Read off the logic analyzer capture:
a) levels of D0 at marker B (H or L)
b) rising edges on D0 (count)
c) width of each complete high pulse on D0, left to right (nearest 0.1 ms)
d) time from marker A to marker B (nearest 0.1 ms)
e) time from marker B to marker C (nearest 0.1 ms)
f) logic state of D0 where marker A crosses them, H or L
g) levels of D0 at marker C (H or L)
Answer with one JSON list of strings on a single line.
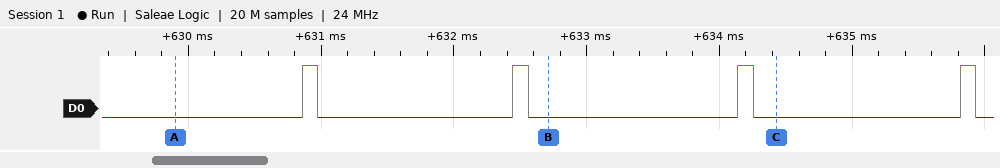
["D0=L", "4", "0.1 ms, 0.1 ms, 0.1 ms, 0.1 ms", "2.8 ms", "1.7 ms", "D0=L", "D0=L"]
